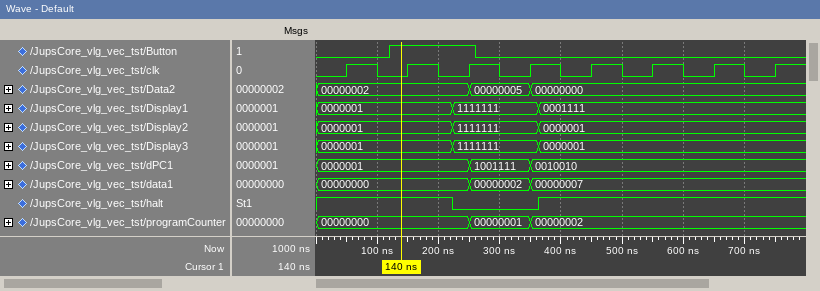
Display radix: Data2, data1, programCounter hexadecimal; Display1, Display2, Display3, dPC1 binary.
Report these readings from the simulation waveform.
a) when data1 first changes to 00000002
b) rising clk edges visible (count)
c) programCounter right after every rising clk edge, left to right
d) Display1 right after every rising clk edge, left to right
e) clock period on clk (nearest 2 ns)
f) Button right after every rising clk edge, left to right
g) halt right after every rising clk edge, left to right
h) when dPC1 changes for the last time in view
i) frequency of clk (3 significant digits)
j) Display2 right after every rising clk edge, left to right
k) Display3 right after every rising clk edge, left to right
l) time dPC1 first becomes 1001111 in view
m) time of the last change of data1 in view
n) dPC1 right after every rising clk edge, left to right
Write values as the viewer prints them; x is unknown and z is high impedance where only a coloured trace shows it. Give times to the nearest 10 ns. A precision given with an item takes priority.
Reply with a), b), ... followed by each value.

a) 250 ns
b) 8
c) 00000000, 00000000, 00000001, 00000002, 00000002, 00000002, 00000002, 00000002
d) 0000001, 0000001, 1111111, 1111111, 0001111, 0001111, 0001111, 0001111
e) 100 ns
f) 0 1 1 0 0 0 0 0
g) 1 1 0 0 1 1 1 1
h) 350 ns
i) 10.0 MHz
j) 0000001, 0000001, 1111111, 1111111, 0000001, 0000001, 0000001, 0000001
k) 0000001, 0000001, 1111111, 1111111, 0000001, 0000001, 0000001, 0000001
l) 250 ns
m) 350 ns
n) 0000001, 0000001, 1001111, 0010010, 0010010, 0010010, 0010010, 0010010
